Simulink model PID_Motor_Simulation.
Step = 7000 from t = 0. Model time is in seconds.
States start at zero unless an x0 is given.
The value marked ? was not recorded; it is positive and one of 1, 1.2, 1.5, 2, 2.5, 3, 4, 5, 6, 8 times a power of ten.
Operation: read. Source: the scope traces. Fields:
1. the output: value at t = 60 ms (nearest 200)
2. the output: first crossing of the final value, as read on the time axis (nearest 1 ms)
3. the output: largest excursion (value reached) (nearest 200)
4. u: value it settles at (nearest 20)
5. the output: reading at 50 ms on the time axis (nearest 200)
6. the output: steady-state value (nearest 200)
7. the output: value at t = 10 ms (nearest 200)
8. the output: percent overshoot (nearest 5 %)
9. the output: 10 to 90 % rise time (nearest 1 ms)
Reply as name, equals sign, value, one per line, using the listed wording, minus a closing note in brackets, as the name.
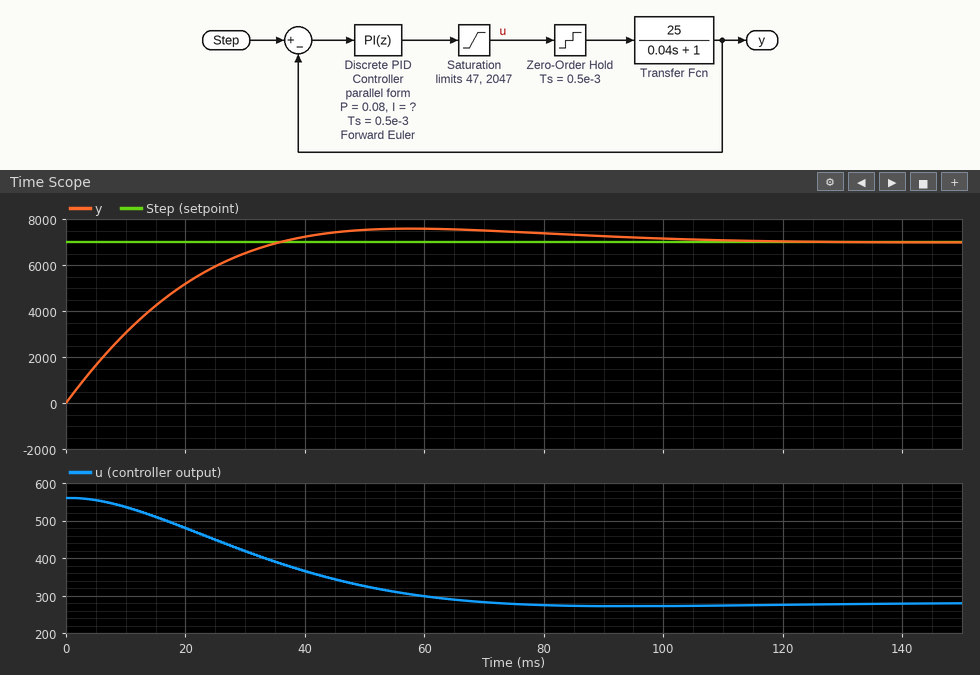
the output: value at t = 60 ms = 7600
the output: first crossing of the final value, as read on the time axis = 36 ms
the output: largest excursion (value reached) = 7600
u: value it settles at = 280
the output: reading at 50 ms on the time axis = 7600
the output: steady-state value = 7000
the output: value at t = 10 ms = 3000
the output: percent overshoot = 10 %
the output: 10 to 90 % rise time = 26 ms
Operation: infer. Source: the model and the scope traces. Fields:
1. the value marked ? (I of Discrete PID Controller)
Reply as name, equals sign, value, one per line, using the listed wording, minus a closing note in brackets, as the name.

the value marked ? = 4
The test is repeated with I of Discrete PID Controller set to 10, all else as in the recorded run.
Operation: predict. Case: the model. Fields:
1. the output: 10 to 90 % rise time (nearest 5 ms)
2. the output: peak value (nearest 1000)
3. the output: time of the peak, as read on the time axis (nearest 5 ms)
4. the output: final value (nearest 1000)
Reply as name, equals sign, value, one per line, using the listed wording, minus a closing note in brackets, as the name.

the output: 10 to 90 % rise time = 15 ms
the output: peak value = 9000
the output: time of the peak, as read on the time axis = 35 ms
the output: final value = 7000
